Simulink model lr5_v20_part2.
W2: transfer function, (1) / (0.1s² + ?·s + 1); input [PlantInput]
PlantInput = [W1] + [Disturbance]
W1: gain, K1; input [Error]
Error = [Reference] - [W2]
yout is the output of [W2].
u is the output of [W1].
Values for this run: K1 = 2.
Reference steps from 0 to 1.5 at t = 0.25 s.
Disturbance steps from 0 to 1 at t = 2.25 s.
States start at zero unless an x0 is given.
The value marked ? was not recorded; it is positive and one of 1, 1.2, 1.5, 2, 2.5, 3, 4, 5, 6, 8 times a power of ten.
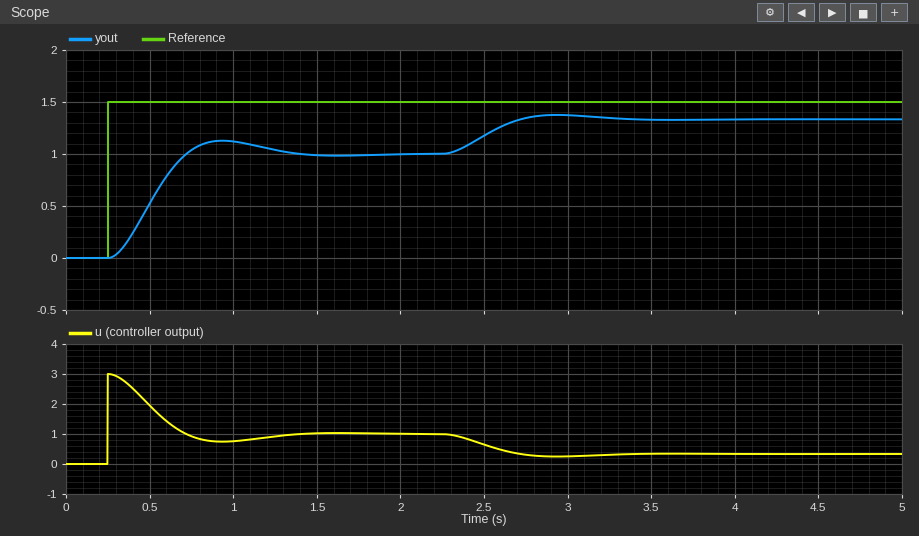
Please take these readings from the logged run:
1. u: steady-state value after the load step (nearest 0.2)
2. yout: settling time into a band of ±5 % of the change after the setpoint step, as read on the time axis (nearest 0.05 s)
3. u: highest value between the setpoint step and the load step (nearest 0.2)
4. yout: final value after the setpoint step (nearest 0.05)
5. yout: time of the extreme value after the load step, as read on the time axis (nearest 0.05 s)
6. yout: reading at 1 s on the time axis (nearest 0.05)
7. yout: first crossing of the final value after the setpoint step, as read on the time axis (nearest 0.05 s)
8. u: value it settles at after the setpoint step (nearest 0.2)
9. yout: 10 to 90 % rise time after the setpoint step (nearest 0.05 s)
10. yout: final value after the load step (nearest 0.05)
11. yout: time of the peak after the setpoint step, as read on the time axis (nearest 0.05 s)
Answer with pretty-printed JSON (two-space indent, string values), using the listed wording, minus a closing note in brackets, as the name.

{
  "u: steady-state value after the load step": "0.4",
  "yout: settling time into a band of ±5 % of the change after the setpoint step, as read on the time axis": "1.20 s",
  "u: highest value between the setpoint step and the load step": "3.0",
  "yout: final value after the setpoint step": "1.00",
  "yout: time of the extreme value after the load step, as read on the time axis": "2.95 s",
  "yout: reading at 1 s on the time axis": "1.10",
  "yout: first crossing of the final value after the setpoint step, as read on the time axis": "0.70 s",
  "u: value it settles at after the setpoint step": "1.0",
  "yout: 10 to 90 % rise time after the setpoint step": "0.30 s",
  "yout: final value after the load step": "1.35",
  "yout: time of the peak after the setpoint step, as read on the time axis": "0.95 s"
}
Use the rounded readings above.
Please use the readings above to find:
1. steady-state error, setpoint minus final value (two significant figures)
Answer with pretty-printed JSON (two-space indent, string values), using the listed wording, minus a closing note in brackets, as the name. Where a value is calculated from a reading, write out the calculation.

{
  "steady-state error, setpoint minus final value": "1.5 - 1 = 0.50"
}
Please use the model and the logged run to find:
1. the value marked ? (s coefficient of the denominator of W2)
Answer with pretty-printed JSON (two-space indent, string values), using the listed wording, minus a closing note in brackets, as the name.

{
  "the value marked ?": "0.6"
}
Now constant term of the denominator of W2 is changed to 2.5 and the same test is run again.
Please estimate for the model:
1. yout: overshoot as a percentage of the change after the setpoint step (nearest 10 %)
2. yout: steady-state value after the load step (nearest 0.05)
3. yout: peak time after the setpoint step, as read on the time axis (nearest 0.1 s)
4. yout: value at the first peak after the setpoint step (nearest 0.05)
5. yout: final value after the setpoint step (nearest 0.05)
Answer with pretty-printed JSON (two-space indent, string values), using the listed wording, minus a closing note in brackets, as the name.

{
  "yout: overshoot as a percentage of the change after the setpoint step": "20 %",
  "yout: steady-state value after the load step": "0.90",
  "yout: peak time after the setpoint step, as read on the time axis": "0.8 s",
  "yout: value at the first peak after the setpoint step": "0.80",
  "yout: final value after the setpoint step": "0.65"
}
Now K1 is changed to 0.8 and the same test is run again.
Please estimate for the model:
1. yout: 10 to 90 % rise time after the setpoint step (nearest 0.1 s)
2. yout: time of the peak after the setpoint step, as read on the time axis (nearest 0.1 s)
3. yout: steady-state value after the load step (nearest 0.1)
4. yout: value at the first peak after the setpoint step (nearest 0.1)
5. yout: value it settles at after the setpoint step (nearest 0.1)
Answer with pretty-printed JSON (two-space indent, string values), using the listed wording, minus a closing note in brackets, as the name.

{
  "yout: 10 to 90 % rise time after the setpoint step": "0.5 s",
  "yout: time of the peak after the setpoint step, as read on the time axis": "1.3 s",
  "yout: steady-state value after the load step": "1.2",
  "yout: value at the first peak after the setpoint step": "0.7",
  "yout: value it settles at after the setpoint step": "0.7"
}
